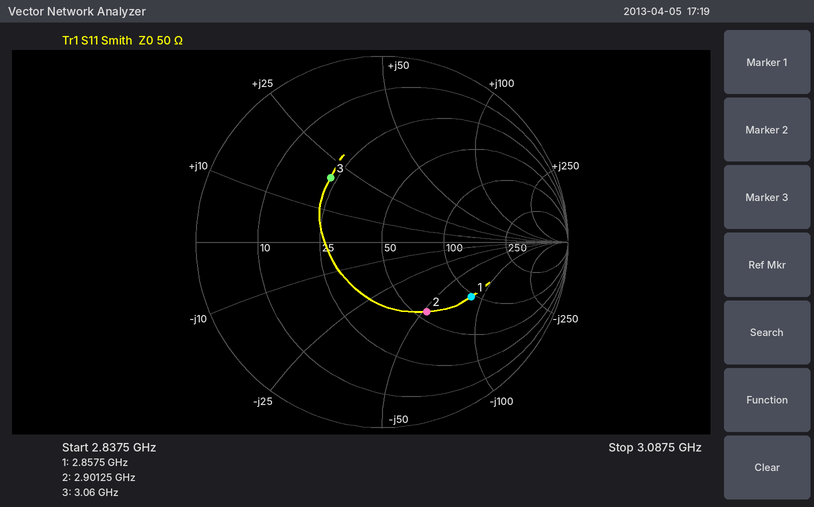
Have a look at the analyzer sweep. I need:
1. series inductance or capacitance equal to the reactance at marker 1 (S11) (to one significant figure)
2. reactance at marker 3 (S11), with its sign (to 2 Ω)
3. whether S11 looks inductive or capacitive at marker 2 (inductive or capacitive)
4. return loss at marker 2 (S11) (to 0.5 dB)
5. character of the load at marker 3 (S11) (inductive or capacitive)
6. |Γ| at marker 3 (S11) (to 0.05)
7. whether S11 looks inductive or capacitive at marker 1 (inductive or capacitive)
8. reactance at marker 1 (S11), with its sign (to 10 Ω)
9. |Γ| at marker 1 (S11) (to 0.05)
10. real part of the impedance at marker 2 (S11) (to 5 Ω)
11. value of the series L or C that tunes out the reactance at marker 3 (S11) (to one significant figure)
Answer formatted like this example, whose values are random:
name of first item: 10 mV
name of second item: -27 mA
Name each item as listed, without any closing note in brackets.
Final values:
series inductance or capacitance equal to the reactance at marker 1 (S11): 700 fF
reactance at marker 3 (S11), with its sign: +20 Ω
whether S11 looks inductive or capacitive at marker 2: capacitive
return loss at marker 2 (S11): 7.0 dB
character of the load at marker 3 (S11): inductive
|Γ| at marker 3 (S11): 0.45
whether S11 looks inductive or capacitive at marker 1: capacitive
reactance at marker 1 (S11), with its sign: -80 Ω
|Γ| at marker 1 (S11): 0.55
real part of the impedance at marker 2 (S11): 55 Ω
value of the series L or C that tunes out the reactance at marker 3 (S11): 3 pF
